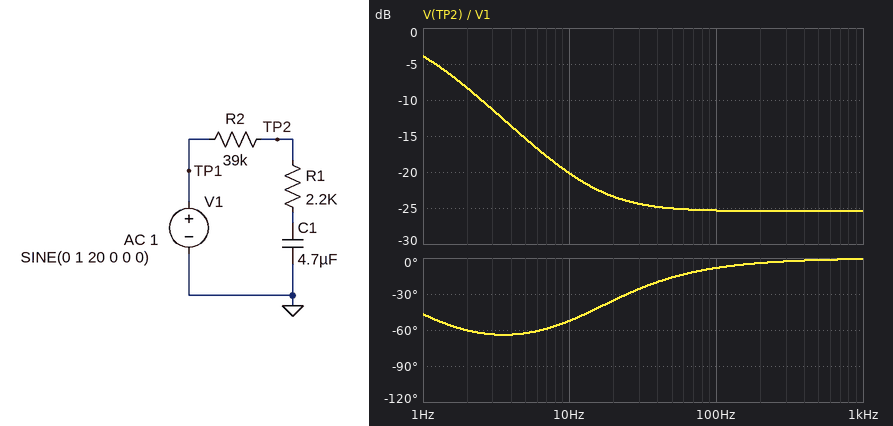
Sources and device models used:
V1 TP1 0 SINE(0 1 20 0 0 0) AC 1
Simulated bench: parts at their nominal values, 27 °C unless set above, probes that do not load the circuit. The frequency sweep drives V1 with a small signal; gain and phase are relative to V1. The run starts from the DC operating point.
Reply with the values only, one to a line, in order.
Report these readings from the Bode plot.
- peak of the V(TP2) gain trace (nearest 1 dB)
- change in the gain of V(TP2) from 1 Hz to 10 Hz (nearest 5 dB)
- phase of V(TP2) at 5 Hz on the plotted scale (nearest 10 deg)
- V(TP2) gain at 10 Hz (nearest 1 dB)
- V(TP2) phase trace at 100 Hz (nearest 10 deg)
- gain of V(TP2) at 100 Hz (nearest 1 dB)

-4 dB
-15 dB
-60 deg
-20 dB
-10 deg
-25 dB
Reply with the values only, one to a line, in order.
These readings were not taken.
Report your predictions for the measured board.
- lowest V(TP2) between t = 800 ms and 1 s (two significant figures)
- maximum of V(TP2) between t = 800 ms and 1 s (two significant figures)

-67 mV
68 mV
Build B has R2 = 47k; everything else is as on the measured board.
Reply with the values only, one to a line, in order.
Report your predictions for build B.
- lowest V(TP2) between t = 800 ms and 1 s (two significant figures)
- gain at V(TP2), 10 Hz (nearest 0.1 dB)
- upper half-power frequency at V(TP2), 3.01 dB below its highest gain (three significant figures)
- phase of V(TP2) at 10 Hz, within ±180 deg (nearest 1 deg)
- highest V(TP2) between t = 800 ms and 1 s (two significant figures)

-56 mV
-21.7 dB
690 mHz
-53 deg
57 mV
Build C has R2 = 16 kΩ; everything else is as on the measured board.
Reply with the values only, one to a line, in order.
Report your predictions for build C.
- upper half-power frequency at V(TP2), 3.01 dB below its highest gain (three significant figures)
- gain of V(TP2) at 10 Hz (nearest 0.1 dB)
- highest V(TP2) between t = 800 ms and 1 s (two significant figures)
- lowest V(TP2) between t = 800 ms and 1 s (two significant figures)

1.89 Hz
-13.2 dB
150 mV
-150 mV
